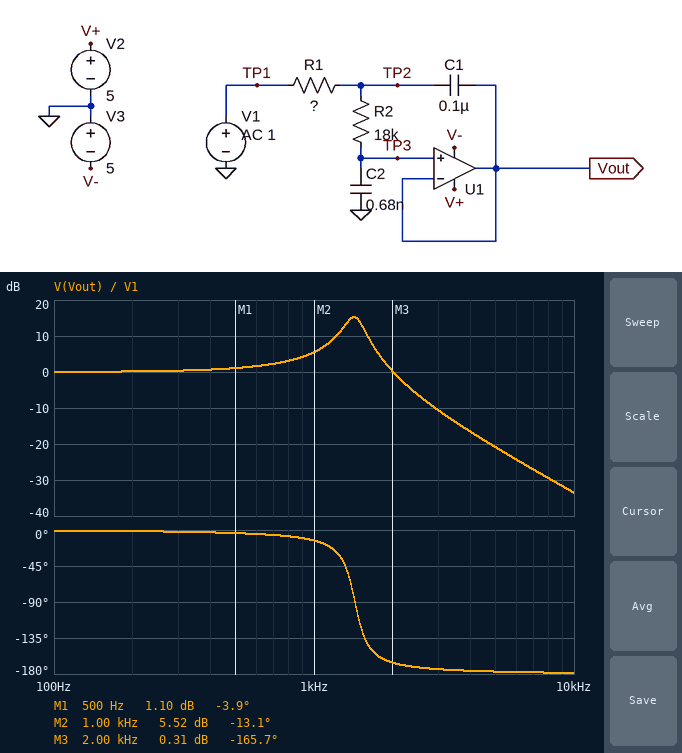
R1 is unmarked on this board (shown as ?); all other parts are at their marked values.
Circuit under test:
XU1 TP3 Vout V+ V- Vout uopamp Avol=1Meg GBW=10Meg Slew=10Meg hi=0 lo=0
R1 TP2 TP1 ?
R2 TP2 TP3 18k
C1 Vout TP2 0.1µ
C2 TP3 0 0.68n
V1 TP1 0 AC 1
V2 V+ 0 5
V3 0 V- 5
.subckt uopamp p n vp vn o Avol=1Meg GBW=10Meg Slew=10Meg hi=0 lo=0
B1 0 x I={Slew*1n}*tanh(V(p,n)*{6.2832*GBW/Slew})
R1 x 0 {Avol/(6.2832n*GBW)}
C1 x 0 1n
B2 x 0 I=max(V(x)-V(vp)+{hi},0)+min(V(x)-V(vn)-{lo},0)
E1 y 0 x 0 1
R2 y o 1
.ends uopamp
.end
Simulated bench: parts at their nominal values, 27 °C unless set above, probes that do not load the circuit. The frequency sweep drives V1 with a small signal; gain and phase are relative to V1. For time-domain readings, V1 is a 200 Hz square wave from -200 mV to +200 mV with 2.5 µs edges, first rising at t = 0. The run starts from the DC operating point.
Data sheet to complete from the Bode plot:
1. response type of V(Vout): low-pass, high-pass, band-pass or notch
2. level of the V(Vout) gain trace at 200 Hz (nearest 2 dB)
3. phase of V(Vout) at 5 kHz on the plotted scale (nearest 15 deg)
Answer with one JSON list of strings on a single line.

["low-pass", "0 dB", "-180 deg"]
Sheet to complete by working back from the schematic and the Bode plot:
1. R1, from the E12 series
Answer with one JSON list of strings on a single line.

["10 kΩ"]
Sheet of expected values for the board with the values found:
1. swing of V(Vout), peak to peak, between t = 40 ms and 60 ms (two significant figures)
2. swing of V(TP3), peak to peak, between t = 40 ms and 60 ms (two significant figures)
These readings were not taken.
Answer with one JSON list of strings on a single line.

["1.1 V", "1.1 V"]
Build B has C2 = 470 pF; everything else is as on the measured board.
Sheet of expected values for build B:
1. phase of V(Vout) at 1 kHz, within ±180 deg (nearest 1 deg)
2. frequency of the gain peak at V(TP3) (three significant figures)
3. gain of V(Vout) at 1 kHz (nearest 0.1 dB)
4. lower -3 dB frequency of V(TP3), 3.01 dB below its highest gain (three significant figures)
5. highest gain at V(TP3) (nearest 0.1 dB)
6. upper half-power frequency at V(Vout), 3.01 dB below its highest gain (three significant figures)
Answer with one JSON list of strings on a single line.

["-7 deg", "1.72 kHz", "3.5 dB", "1.59 kHz", "16.9 dB", "1.84 kHz"]
